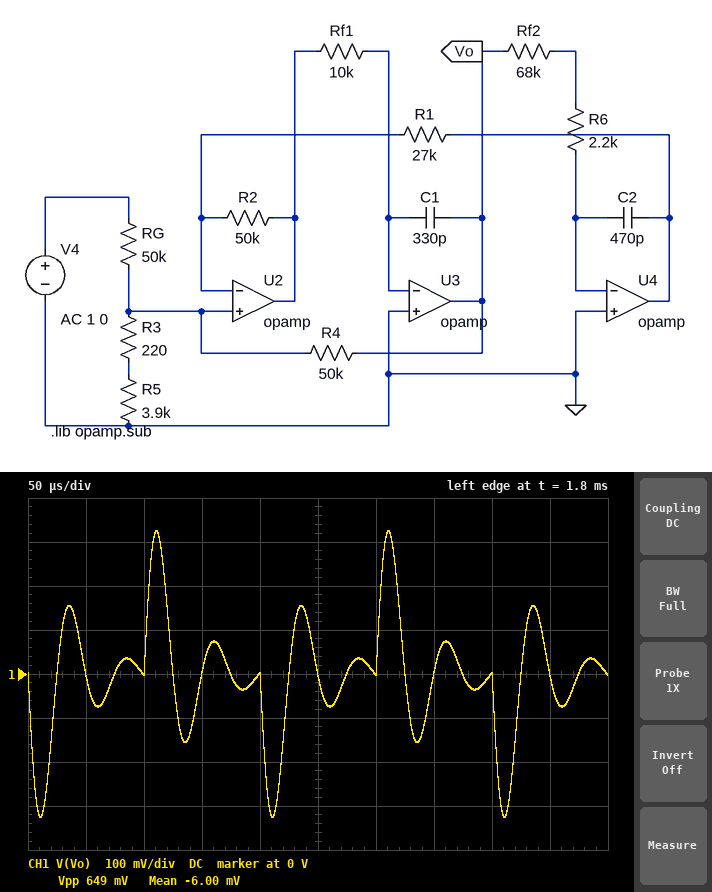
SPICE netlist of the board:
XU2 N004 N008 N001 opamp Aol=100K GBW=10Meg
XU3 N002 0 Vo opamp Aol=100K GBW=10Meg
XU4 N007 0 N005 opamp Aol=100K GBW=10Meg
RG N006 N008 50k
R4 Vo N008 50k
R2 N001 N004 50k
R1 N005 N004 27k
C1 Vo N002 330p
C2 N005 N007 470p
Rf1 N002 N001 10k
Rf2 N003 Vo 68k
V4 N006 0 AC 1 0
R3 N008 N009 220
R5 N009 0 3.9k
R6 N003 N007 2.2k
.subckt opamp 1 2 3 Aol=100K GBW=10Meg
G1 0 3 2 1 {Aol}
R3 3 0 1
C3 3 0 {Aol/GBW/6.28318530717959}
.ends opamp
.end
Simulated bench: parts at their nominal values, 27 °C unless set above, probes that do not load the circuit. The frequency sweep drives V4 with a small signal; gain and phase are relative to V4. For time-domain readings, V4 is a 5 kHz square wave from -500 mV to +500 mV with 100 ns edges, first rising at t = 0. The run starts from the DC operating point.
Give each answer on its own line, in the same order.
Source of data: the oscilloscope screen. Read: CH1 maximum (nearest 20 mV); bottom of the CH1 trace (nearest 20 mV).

320 mV
-320 mV
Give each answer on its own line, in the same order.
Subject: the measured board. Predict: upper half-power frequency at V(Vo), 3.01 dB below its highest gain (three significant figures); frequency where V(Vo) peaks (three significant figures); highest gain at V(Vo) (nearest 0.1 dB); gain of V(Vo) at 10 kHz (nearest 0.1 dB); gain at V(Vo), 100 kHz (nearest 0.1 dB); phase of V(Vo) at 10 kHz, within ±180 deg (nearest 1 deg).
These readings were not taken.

26.0 kHz
20.7 kHz
0.2 dB
-11.0 dB
-19.9 dB
-106 deg
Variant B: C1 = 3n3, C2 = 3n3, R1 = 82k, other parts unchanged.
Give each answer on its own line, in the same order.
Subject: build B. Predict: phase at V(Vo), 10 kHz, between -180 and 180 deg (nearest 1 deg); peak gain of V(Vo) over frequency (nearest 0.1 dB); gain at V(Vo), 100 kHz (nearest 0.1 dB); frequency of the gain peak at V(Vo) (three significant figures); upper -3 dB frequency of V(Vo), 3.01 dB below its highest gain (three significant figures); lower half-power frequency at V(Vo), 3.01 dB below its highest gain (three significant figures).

93 deg
0 dB
-45.2 dB
1.42 kHz
1.72 kHz
1.17 kHz
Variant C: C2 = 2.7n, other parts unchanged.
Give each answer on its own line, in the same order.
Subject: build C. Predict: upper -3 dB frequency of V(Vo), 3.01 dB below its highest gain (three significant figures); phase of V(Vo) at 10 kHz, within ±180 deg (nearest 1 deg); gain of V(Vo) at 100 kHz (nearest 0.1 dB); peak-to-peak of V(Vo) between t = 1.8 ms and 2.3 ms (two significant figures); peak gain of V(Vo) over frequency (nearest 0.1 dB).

14.8 kHz
165 deg
-20.2 dB
1.2 V
0 dB
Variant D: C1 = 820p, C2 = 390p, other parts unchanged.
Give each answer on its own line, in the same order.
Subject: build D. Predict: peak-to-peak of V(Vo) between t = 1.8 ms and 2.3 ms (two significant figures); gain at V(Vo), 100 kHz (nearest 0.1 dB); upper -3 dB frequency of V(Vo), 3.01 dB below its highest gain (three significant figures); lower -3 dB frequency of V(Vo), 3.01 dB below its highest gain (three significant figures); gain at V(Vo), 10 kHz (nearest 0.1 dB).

590 mV
-28.0 dB
16.5 kHz
12.7 kHz
-9.4 dB
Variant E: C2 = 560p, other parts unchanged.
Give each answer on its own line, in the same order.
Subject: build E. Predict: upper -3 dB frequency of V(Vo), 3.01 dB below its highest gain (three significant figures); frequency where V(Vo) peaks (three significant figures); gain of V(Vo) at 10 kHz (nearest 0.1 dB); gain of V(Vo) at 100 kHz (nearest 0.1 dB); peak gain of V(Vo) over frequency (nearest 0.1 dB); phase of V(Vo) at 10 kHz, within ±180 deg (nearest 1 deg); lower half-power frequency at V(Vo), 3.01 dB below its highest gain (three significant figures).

24.4 kHz
19.0 kHz
-9.1 dB
-20.0 dB
0.2 dB
-110 deg
14.8 kHz
